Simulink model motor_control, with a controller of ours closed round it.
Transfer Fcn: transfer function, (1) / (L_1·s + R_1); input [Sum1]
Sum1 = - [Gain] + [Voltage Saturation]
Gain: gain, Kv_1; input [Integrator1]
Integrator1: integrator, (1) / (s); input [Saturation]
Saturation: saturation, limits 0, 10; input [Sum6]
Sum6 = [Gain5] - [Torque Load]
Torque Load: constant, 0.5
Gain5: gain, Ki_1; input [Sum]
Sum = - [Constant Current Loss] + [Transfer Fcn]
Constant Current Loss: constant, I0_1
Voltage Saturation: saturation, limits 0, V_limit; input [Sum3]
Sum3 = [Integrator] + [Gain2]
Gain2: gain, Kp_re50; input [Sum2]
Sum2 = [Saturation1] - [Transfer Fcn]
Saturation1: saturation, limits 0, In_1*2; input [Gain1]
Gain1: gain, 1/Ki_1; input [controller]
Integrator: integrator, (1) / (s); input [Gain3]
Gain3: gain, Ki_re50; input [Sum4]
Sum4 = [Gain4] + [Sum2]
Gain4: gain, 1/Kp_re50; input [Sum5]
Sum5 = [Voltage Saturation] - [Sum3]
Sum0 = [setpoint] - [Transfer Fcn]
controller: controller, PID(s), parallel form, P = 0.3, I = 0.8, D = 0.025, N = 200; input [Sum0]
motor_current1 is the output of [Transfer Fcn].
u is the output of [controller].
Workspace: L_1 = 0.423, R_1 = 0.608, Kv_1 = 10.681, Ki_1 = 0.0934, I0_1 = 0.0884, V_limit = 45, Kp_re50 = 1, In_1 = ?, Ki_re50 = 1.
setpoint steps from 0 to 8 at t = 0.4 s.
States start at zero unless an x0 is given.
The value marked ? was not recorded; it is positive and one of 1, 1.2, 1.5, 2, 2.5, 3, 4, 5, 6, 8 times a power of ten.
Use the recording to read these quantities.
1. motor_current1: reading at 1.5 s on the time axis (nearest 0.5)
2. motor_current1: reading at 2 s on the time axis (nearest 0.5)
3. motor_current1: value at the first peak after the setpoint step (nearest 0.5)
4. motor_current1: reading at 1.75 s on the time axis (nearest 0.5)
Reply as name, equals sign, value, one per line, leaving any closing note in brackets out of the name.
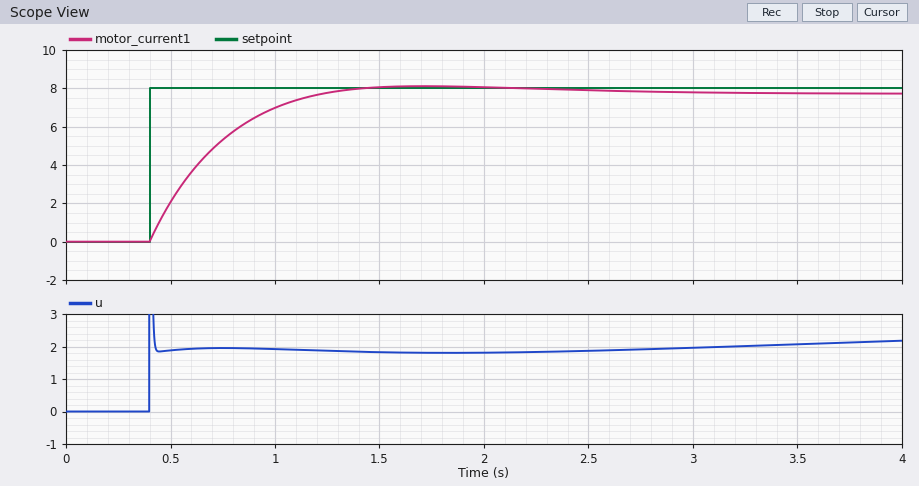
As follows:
motor_current1: reading at 1.5 s on the time axis = 8.0
motor_current1: reading at 2 s on the time axis = 8.0
motor_current1: value at the first peak after the setpoint step = 8.0
motor_current1: reading at 1.75 s on the time axis = 8.0
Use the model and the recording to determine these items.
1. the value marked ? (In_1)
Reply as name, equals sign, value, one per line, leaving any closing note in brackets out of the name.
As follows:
the value marked ? = 5
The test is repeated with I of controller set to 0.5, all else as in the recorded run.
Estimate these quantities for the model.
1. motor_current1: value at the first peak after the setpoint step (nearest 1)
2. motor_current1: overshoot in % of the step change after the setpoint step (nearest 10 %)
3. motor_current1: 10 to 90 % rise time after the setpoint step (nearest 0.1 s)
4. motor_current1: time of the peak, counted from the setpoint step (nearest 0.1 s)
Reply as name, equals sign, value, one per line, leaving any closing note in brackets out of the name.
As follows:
motor_current1: value at the first peak after the setpoint step = 8
motor_current1: overshoot in % of the step change after the setpoint step = 50 %
motor_current1: 10 to 90 % rise time after the setpoint step = 0.3 s
motor_current1: time of the peak, counted from the setpoint step = 1.3 s
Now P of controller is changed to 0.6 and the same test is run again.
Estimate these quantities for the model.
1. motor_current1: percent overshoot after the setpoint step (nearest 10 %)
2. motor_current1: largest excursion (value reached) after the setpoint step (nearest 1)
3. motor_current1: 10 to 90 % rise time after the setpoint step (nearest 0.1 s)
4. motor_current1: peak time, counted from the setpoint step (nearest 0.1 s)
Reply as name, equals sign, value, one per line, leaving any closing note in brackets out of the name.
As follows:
motor_current1: percent overshoot after the setpoint step = 50 %
motor_current1: largest excursion (value reached) after the setpoint step = 8
motor_current1: 10 to 90 % rise time after the setpoint step = 0.3 s
motor_current1: peak time, counted from the setpoint step = 1.3 s
